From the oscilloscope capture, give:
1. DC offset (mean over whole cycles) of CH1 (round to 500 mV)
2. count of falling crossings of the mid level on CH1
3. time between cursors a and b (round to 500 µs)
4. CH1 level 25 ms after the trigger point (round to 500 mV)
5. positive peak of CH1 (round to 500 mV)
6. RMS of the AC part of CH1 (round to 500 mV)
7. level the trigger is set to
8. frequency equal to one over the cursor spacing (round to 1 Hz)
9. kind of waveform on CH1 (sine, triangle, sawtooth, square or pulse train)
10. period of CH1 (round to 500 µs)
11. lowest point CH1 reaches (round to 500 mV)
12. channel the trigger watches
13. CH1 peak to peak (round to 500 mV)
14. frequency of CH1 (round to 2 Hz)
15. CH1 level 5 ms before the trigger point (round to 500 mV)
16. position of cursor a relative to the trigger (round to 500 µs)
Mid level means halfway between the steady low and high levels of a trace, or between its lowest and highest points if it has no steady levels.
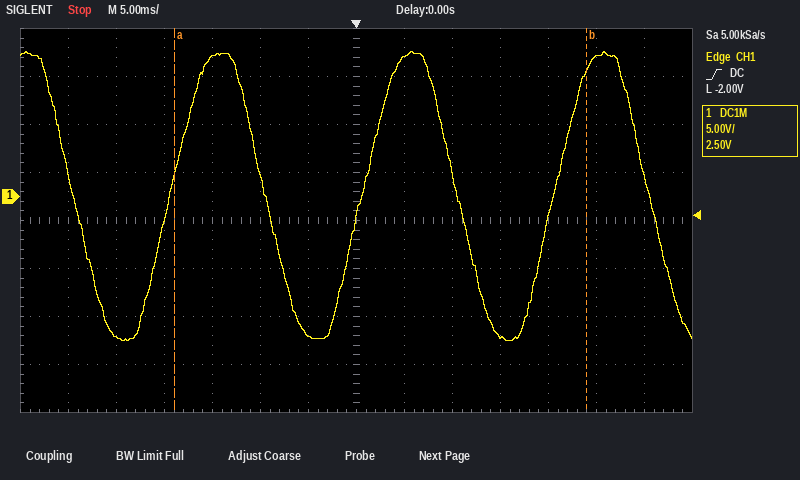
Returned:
0.0 V
4
43.0 ms
14.5 V
15.0 V
10.5 V
-2.00 V
23 Hz
sine
20.0 ms
-15.0 V
CH1
30.0 V
50 Hz
-14.5 V
-19.0 ms
